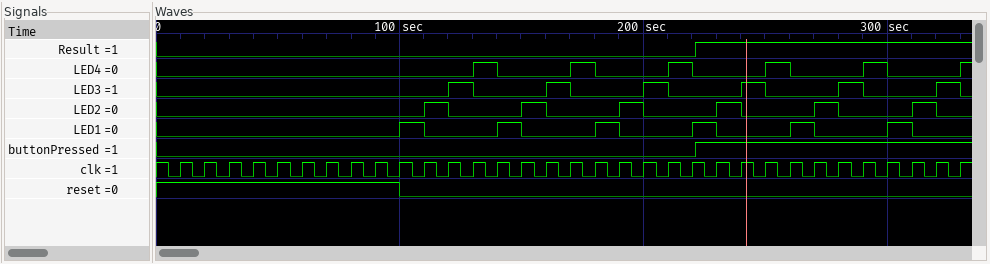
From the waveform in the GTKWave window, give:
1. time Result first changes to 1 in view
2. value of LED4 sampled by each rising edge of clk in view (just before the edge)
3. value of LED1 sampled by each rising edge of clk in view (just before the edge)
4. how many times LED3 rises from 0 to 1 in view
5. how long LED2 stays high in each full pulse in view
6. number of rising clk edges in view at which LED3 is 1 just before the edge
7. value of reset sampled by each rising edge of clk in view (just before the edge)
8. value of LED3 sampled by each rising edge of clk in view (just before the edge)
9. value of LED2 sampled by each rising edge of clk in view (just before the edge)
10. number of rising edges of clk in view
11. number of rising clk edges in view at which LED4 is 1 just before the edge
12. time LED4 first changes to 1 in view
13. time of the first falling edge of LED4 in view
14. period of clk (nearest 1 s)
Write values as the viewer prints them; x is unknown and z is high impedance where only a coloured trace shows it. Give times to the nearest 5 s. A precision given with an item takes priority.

220 s
0 0 0 0 0 0 0 0 0 0 0 0 0 1 0 0 0 1 0 0 0 1 0 0 0 1 0 0 0 1 0 0 0
0 0 0 0 0 0 0 0 0 0 1 0 0 0 1 0 0 0 1 0 0 0 1 0 0 0 1 0 0 0 1 0 0
6
10 s, 10 s, 10 s, 10 s, 10 s, 10 s
6
1 1 1 1 1 1 1 1 1 1 0 0 0 0 0 0 0 0 0 0 0 0 0 0 0 0 0 0 0 0 0 0 0
0 0 0 0 0 0 0 0 0 0 0 0 1 0 0 0 1 0 0 0 1 0 0 0 1 0 0 0 1 0 0 0 1
0 0 0 0 0 0 0 0 0 0 0 1 0 0 0 1 0 0 0 1 0 0 0 1 0 0 0 1 0 0 0 1 0
33
5
130 s
140 s
10 s
